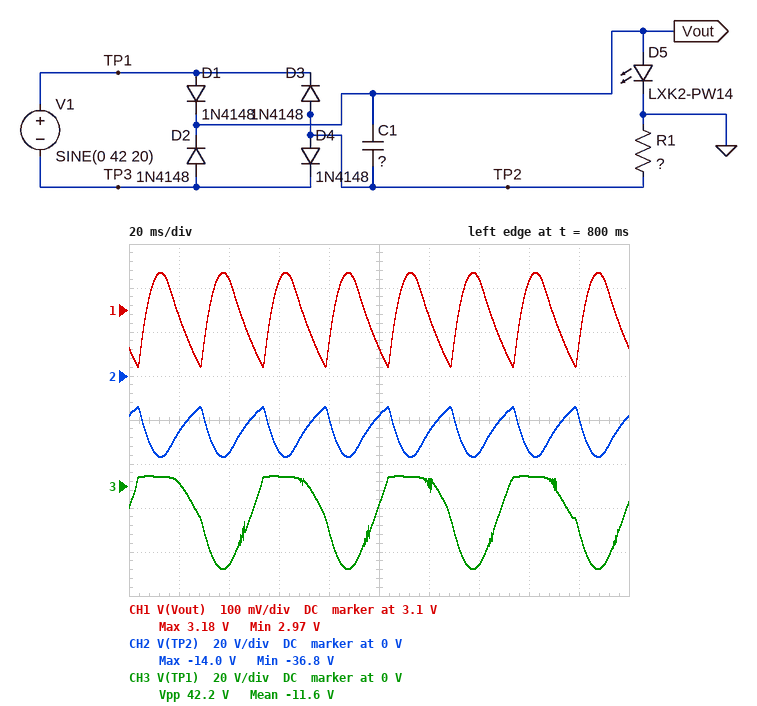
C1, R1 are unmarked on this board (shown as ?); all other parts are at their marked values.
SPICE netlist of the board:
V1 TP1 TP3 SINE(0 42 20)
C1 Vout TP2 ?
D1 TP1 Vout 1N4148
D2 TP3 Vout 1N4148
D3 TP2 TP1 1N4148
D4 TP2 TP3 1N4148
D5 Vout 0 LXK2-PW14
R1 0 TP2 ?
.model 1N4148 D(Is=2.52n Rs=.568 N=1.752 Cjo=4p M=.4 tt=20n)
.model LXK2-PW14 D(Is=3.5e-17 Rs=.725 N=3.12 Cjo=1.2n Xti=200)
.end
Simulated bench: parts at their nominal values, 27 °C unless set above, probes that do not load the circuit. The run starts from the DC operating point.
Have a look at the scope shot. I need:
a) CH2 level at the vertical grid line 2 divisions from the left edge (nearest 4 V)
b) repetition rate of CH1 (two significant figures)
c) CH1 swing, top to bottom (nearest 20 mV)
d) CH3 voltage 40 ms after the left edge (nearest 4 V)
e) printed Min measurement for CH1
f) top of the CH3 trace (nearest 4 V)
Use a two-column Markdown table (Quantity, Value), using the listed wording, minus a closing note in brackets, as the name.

| Quantity | Value |
|---|---|
| CH2 level at the vertical grid line 2 divisions from the left edge | -36 V |
| repetition rate of CH1 | 40 Hz |
| CH1 swing, top to bottom | 220 mV |
| CH3 voltage 40 ms after the left edge | -36 V |
| printed Min measurement for CH1 | 2.97 V |
| top of the CH3 trace | 4 V |
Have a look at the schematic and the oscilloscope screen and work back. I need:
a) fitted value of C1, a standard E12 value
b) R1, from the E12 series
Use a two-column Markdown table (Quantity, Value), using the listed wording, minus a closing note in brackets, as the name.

| Quantity | Value |
|---|---|
| fitted value of C1, a standard E12 value | 120 µF |
| R1, from the E12 series | 120 Ω |
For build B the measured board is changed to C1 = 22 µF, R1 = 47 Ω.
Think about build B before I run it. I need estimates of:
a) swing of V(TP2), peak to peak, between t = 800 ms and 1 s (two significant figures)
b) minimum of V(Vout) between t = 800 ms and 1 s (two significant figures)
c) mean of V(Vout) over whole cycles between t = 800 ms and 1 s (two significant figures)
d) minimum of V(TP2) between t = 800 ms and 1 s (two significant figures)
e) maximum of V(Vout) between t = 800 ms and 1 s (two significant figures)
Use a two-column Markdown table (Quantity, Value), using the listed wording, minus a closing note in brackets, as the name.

| Quantity | Value |
|---|---|
| swing of V(TP2), peak to peak, between t = 800 ms and 1 s | 35 V |
| minimum of V(Vout) between t = 800 ms and 1 s | 2.7 V |
| mean of V(Vout) over whole cycles between t = 800 ms and 1 s | 3.3 V |
| minimum of V(TP2) between t = 800 ms and 1 s | -36 V |
| maximum of V(Vout) between t = 800 ms and 1 s | 3.6 V |
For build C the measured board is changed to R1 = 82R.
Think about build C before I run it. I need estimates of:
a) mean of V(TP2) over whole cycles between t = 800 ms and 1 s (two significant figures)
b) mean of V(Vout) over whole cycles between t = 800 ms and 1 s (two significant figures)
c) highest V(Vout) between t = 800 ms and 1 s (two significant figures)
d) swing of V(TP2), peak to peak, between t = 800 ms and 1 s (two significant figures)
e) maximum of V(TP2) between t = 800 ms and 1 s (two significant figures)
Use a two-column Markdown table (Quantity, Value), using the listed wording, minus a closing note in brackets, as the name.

| Quantity | Value |
|---|---|
| mean of V(TP2) over whole cycles between t = 800 ms and 1 s | -25 V |
| mean of V(Vout) over whole cycles between t = 800 ms and 1 s | 3.2 V |
| highest V(Vout) between t = 800 ms and 1 s | 3.3 V |
| swing of V(TP2), peak to peak, between t = 800 ms and 1 s | 26 V |
| maximum of V(TP2) between t = 800 ms and 1 s | -10 V |
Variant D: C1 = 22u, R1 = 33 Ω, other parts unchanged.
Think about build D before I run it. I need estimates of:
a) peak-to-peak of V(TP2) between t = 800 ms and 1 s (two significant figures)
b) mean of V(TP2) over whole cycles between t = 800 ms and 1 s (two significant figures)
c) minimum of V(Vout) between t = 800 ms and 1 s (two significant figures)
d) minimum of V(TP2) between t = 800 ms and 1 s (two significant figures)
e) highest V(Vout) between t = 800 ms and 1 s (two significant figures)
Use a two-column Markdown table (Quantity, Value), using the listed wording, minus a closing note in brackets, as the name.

| Quantity | Value |
|---|---|
| peak-to-peak of V(TP2) between t = 800 ms and 1 s | 35 V |
| mean of V(TP2) over whole cycles between t = 800 ms and 1 s | -21 V |
| minimum of V(Vout) between t = 800 ms and 1 s | 2.7 V |
| minimum of V(TP2) between t = 800 ms and 1 s | -35 V |
| highest V(Vout) between t = 800 ms and 1 s | 3.8 V |
